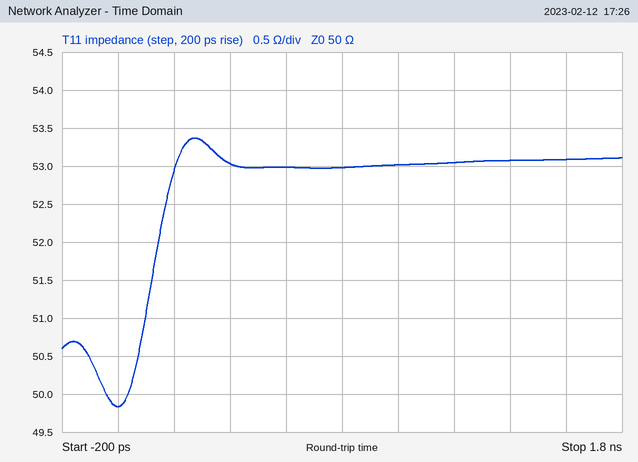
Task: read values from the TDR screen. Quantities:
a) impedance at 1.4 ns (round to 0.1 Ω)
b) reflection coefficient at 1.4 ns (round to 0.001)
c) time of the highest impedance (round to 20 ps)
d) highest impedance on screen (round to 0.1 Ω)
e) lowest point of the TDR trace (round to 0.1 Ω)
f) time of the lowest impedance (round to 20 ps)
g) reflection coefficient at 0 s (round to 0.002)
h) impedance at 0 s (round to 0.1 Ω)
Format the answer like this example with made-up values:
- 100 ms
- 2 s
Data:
- 53.1 Ω
- +0.030
- 280 ps
- 53.4 Ω
- 49.8 Ω
- 0 ps
- -0.002
- 49.8 Ω
